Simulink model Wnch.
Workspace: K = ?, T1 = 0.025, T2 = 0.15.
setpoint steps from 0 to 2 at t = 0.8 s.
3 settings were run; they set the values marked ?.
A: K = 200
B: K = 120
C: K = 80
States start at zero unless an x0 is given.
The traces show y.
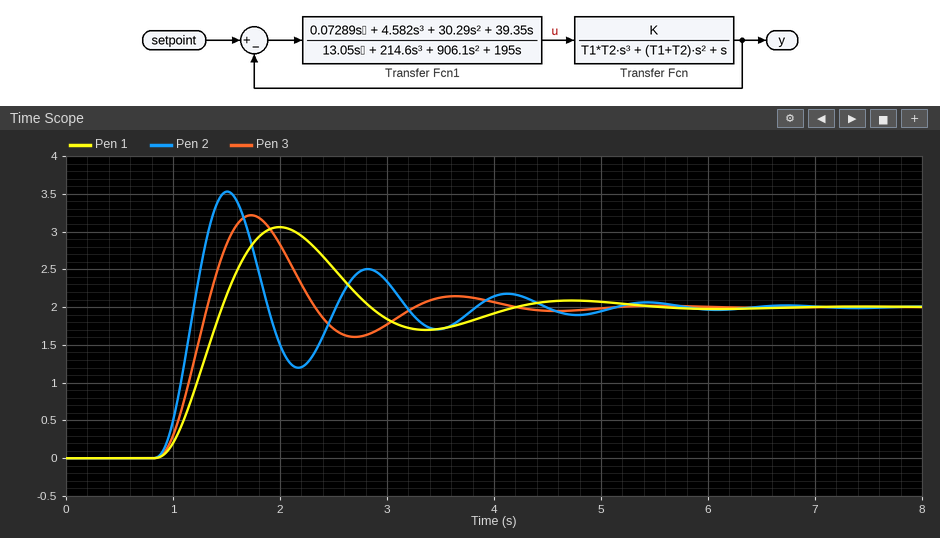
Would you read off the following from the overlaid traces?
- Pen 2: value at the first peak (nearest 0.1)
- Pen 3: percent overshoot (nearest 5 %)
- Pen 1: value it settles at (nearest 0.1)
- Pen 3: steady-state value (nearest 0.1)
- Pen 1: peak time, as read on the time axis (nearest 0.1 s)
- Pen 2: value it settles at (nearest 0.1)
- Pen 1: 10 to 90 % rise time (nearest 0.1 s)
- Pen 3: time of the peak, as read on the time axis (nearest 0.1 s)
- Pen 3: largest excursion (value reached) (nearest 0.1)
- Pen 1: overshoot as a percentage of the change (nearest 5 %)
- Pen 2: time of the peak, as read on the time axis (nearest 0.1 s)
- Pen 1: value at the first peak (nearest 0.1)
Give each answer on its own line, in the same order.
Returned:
3.5
60 %
2.0
2.0
2.0 s
2.0
0.4 s
1.7 s
3.2
55 %
1.5 s
3.1
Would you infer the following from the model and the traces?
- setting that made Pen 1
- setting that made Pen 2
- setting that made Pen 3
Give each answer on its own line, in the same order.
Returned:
C
A
B
